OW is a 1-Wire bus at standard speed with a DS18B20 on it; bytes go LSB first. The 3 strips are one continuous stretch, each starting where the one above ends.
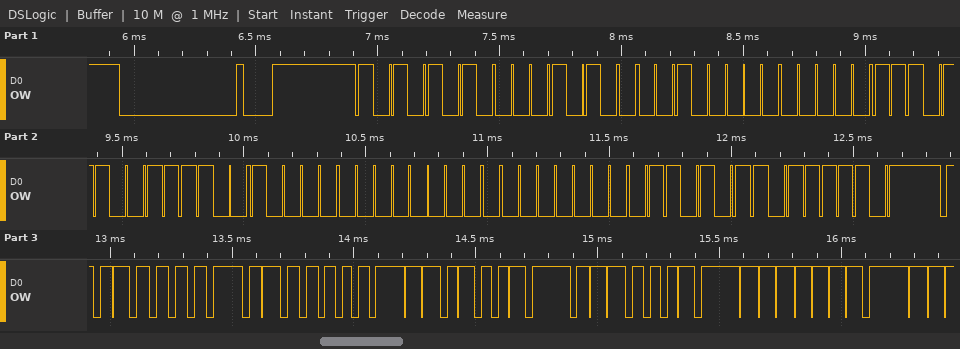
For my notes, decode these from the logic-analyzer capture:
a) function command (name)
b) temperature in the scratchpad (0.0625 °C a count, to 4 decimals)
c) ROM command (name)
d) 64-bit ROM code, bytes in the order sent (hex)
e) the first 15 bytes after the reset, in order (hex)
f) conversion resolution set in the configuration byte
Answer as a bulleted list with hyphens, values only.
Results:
- Read Scratchpad
- 32.2500 °C
- Match ROM
- 28 04 E0 E6 09 00 00 D6
- 55 28 04 E0 E6 09 00 00 D6 BE 04 02 4B 46 7F
- 12 bits
